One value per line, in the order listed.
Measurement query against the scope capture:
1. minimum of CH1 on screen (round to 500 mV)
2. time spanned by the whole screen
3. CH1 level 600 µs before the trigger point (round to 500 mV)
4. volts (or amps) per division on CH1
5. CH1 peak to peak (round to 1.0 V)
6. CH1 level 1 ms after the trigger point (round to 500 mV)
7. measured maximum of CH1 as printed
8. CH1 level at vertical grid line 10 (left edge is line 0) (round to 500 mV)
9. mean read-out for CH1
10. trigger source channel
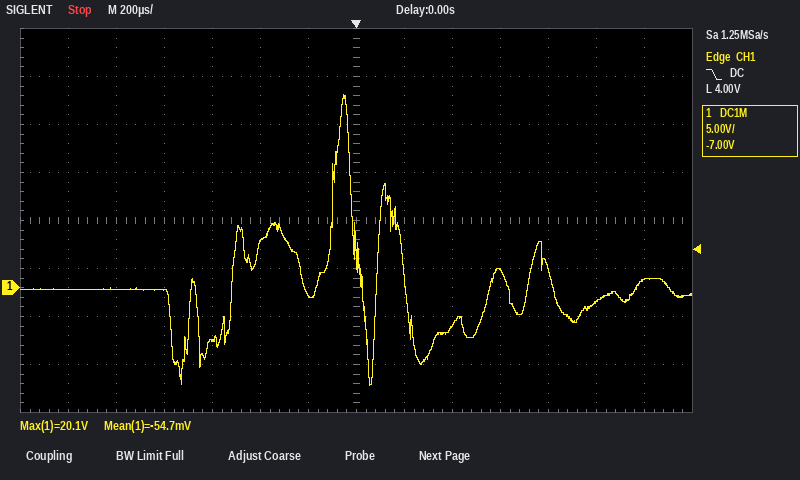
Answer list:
-10.0 V
2.8 ms
-5.5 V
5 V
30.0 V
-1.5 V
20.1 V
2.0 V
-54.7 mV
CH1
